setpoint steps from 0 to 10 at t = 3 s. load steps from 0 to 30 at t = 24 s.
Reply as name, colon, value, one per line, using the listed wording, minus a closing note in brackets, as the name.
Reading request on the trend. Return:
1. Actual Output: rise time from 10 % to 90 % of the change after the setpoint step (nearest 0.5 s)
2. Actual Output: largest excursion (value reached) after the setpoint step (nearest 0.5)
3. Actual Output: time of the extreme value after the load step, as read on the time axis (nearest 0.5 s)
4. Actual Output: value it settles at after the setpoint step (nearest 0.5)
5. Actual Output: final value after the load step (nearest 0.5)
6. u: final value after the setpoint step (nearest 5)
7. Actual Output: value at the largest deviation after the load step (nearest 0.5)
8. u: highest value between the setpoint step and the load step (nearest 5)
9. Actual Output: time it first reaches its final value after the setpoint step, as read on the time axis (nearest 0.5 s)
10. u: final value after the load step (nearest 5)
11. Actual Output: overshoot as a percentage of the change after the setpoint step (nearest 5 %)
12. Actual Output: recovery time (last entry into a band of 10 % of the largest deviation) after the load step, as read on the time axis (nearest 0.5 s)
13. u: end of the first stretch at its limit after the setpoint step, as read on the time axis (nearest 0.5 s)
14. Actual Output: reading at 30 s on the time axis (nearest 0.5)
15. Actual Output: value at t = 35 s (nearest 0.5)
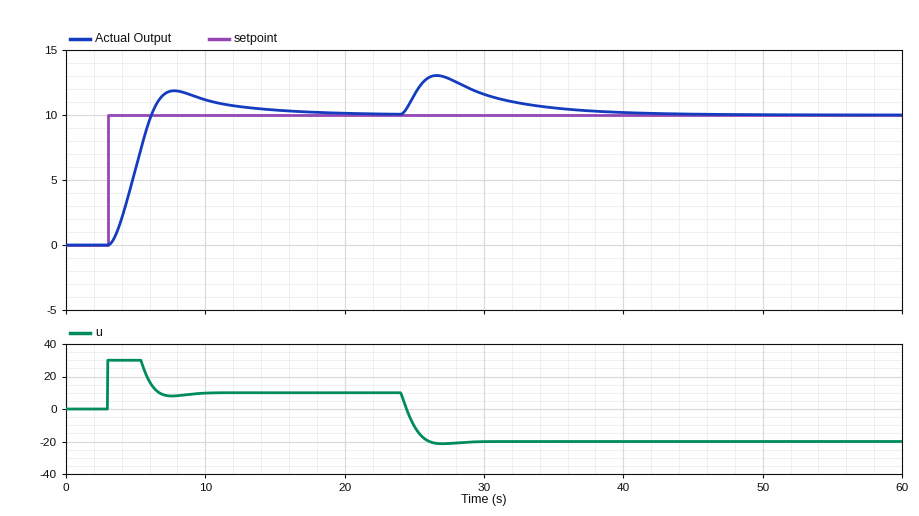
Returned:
Actual Output: rise time from 10 % to 90 % of the change after the setpoint step: 2.0 s
Actual Output: largest excursion (value reached) after the setpoint step: 12.0
Actual Output: time of the extreme value after the load step, as read on the time axis: 26.5 s
Actual Output: value it settles at after the setpoint step: 10.0
Actual Output: final value after the load step: 10.0
u: final value after the setpoint step: 10
Actual Output: value at the largest deviation after the load step: 13.0
u: highest value between the setpoint step and the load step: 30
Actual Output: time it first reaches its final value after the setpoint step, as read on the time axis: 6.0 s
u: final value after the load step: -20
Actual Output: overshoot as a percentage of the change after the setpoint step: 20 %
Actual Output: recovery time (last entry into a band of 10 % of the largest deviation) after the load step, as read on the time axis: 38.0 s
u: end of the first stretch at its limit after the setpoint step, as read on the time axis: 5.5 s
Actual Output: reading at 30 s on the time axis: 11.5
Actual Output: value at t = 35 s: 10.5
